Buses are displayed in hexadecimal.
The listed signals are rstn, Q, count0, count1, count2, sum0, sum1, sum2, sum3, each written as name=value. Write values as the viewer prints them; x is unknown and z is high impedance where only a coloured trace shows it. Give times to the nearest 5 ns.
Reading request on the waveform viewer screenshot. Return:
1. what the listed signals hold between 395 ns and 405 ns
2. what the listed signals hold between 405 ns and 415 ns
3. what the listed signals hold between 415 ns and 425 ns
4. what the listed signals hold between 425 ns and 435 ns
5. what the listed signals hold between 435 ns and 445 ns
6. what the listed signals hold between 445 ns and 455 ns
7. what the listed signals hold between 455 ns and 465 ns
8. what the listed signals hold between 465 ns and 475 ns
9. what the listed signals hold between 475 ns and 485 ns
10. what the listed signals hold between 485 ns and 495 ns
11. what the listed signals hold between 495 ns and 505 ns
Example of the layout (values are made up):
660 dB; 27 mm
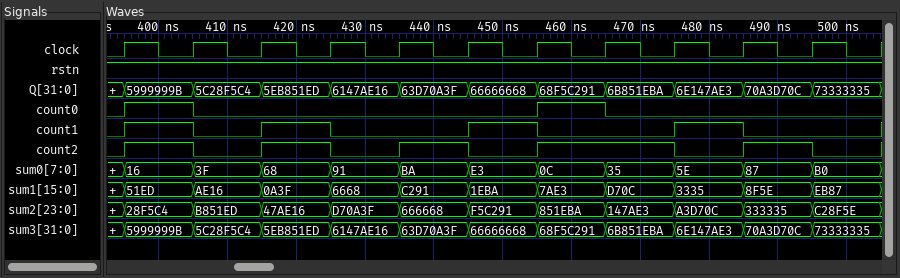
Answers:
rstn=1, Q=5999999B, count0=1, count1=1, count2=1, sum0=16, sum1=51ED, sum2=28F5C4, sum3=5999999B; rstn=1, Q=5C28F5C4, count0=0, count1=0, count2=0, sum0=3F, sum1=AE16, sum2=B851ED, sum3=5C28F5C4; rstn=1, Q=5EB851ED, count0=0, count1=1, count2=1, sum0=68, sum1=0A3F, sum2=47AE16, sum3=5EB851ED; rstn=1, Q=6147AE16, count0=0, count1=0, count2=0, sum0=91, sum1=6668, sum2=D70A3F, sum3=6147AE16; rstn=1, Q=63D70A3F, count0=0, count1=0, count2=1, sum0=BA, sum1=C291, sum2=666668, sum3=63D70A3F; rstn=1, Q=66666668, count0=0, count1=1, count2=0, sum0=E3, sum1=1EBA, sum2=F5C291, sum3=66666668; rstn=1, Q=68F5C291, count0=1, count1=0, count2=1, sum0=0C, sum1=7AE3, sum2=851EBA, sum3=68F5C291; rstn=1, Q=6B851EBA, count0=0, count1=0, count2=1, sum0=35, sum1=D70C, sum2=147AE3, sum3=6B851EBA; rstn=1, Q=6E147AE3, count0=0, count1=1, count2=0, sum0=5E, sum1=3335, sum2=A3D70C, sum3=6E147AE3; rstn=1, Q=70A3D70C, count0=0, count1=0, count2=1, sum0=87, sum1=8F5E, sum2=333335, sum3=70A3D70C; rstn=1, Q=73333335, count0=0, count1=0, count2=0, sum0=B0, sum1=EB87, sum2=C28F5E, sum3=73333335
